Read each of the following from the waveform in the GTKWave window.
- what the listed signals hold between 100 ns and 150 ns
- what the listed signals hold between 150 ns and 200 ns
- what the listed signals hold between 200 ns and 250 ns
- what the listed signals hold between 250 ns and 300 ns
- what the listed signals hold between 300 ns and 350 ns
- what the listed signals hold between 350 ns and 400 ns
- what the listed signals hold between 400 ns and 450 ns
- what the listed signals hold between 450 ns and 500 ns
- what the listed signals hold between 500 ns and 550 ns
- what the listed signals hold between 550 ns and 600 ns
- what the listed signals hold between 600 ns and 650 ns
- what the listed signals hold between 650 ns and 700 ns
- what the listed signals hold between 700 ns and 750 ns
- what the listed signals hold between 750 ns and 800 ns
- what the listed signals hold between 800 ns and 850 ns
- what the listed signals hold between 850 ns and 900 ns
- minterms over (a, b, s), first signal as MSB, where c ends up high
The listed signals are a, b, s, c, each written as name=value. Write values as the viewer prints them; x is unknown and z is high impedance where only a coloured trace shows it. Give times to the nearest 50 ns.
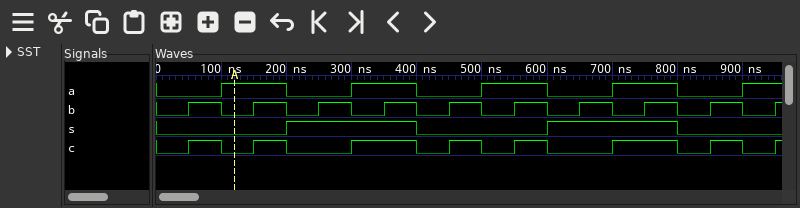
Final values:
a=1, b=0, s=0, c=0
a=1, b=1, s=0, c=1
a=0, b=0, s=1, c=0
a=0, b=1, s=1, c=0
a=1, b=0, s=1, c=1
a=1, b=1, s=1, c=1
a=0, b=0, s=0, c=0
a=0, b=1, s=0, c=1
a=1, b=0, s=0, c=0
a=1, b=1, s=0, c=1
a=0, b=0, s=1, c=0
a=0, b=1, s=1, c=0
a=1, b=0, s=1, c=1
a=1, b=1, s=1, c=1
a=0, b=0, s=0, c=0
a=0, b=1, s=0, c=1
2, 5, 6, 7
